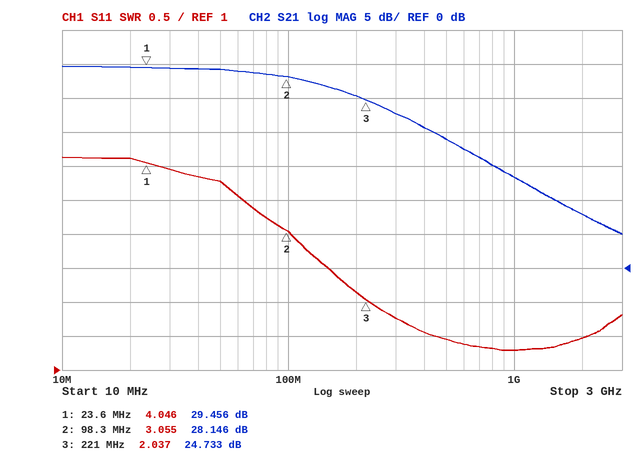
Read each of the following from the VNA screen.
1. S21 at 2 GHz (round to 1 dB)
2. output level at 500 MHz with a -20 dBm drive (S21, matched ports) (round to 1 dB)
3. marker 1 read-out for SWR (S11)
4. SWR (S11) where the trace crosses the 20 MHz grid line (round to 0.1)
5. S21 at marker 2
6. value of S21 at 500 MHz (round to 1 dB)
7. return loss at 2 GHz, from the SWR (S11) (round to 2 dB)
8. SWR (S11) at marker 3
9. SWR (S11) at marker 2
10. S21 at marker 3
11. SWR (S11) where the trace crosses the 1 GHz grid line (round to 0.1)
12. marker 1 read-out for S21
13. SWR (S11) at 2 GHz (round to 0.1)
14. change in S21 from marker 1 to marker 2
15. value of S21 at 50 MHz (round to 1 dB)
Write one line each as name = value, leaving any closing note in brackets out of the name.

S21 at 2 GHz = 8 dB
output level at 500 MHz with a -20 dBm drive (S21, matched ports) = -1 dBm
marker 1 read-out for SWR = 4.046
SWR (S11) where the trace crosses the 20 MHz grid line = 4.1
S21 at marker 2 = 28.146 dB
value of S21 at 500 MHz = 19 dB
return loss at 2 GHz, from the SWR (S11) = 14 dB
SWR (S11) at marker 3 = 2.037
SWR (S11) at marker 2 = 3.055
S21 at marker 3 = 24.733 dB
SWR (S11) where the trace crosses the 1 GHz grid line = 1.3
marker 1 read-out for S21 = 29.456 dB
SWR (S11) at 2 GHz = 1.5
change in S21 from marker 1 to marker 2 = -1.310 dB
value of S21 at 50 MHz = 29 dB
